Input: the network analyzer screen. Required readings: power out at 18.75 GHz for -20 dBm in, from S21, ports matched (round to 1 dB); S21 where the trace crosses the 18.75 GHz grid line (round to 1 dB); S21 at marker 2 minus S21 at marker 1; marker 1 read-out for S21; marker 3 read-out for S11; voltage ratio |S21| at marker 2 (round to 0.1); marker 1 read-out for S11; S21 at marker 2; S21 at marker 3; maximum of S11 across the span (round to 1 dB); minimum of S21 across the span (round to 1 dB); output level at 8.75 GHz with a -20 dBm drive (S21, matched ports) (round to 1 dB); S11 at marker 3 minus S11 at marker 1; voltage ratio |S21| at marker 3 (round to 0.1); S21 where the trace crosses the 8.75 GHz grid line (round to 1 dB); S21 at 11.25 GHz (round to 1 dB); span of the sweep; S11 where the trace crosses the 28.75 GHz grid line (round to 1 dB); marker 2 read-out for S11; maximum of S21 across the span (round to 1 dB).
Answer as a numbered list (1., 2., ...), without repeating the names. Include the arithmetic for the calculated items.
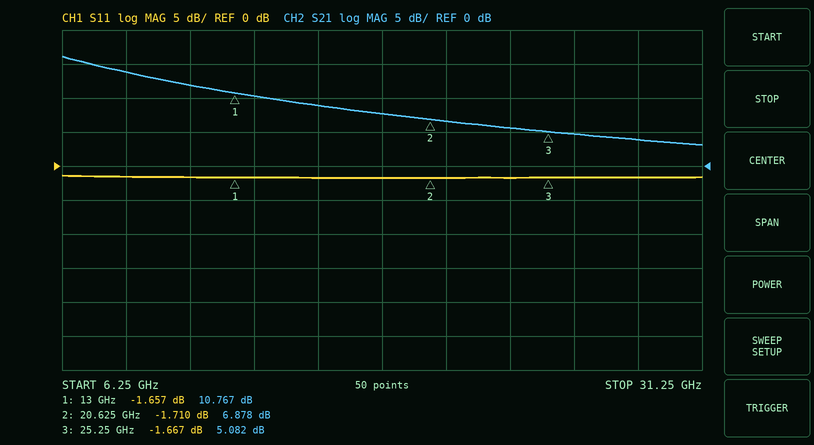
1. -20 dBm + (8 dB) = -12 dBm
2. 8 dB
3. 6.878 − (10.767) = -3.889 dB
4. 10.767 dB
5. -1.667 dB
6. 10^(6.878/20) ≈ 2.2
7. -1.657 dB
8. 6.878 dB
9. 5.082 dB
10. -1 dB
11. 3 dB
12. -20 dBm + (14 dB) = -6 dBm
13. -1.667 − (-1.657) = -0.010 dB
14. 10^(5.082/20) ≈ 1.8
15. 14 dB
16. 12 dB
17. 25 GHz
18. -2 dB
19. -1.710 dB
20. 16 dB
